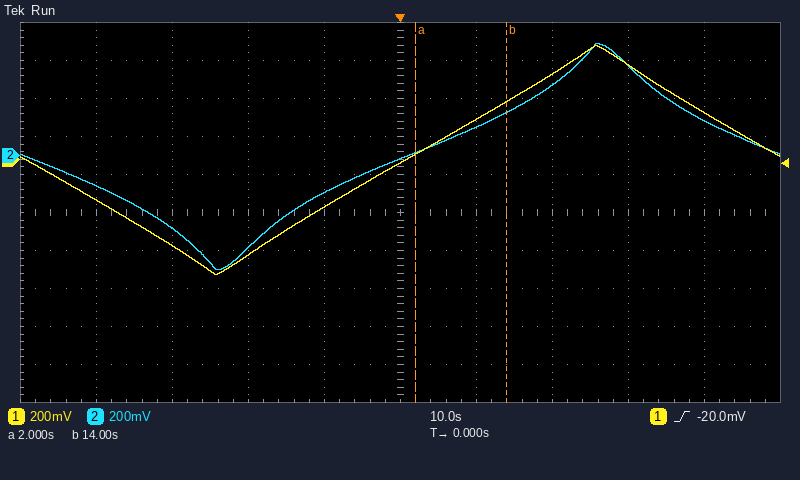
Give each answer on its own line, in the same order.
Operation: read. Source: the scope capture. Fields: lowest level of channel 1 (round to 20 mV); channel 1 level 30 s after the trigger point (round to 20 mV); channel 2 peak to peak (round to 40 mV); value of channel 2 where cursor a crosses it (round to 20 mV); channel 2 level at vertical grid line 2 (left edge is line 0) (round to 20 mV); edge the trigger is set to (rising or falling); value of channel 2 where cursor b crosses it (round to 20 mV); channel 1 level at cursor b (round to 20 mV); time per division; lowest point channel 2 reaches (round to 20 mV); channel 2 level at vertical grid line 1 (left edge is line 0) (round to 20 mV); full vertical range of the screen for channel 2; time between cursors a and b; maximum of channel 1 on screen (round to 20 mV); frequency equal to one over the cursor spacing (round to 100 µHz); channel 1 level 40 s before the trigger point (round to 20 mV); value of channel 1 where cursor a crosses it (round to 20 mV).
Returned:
-600 mV
500 mV
1.20 V
20 mV
-380 mV
rising
220 mV
300 mV
10 s
-600 mV
-160 mV
2 V
12 s
600 mV
83.3 mHz
-220 mV
20 mV
